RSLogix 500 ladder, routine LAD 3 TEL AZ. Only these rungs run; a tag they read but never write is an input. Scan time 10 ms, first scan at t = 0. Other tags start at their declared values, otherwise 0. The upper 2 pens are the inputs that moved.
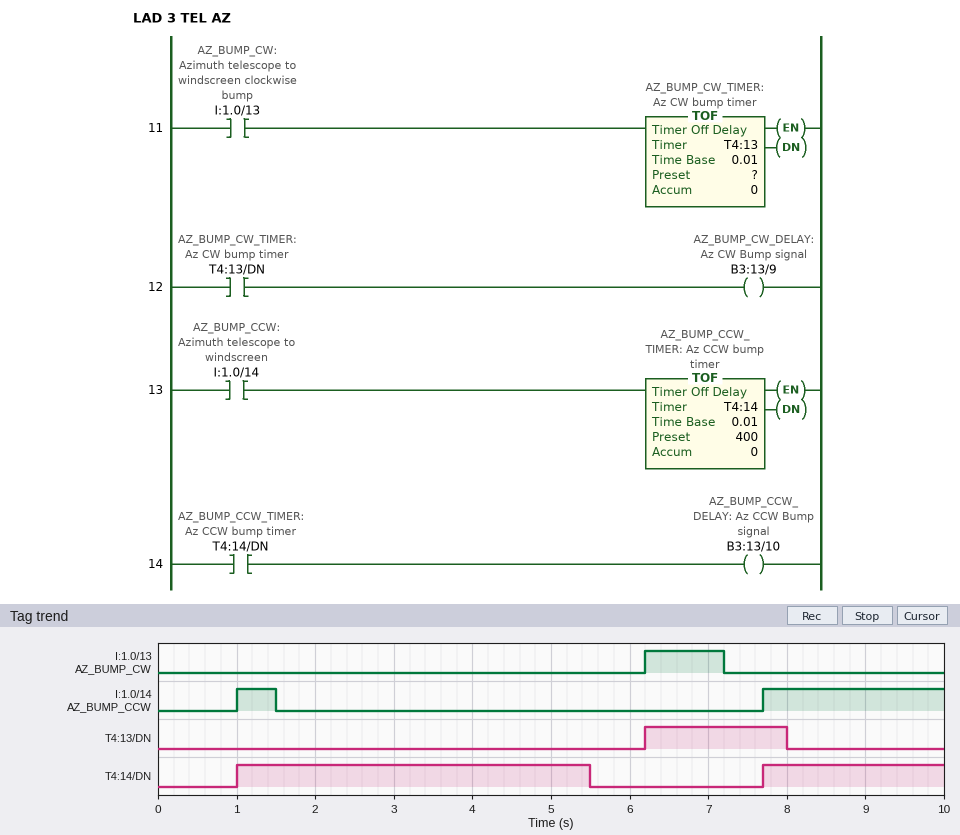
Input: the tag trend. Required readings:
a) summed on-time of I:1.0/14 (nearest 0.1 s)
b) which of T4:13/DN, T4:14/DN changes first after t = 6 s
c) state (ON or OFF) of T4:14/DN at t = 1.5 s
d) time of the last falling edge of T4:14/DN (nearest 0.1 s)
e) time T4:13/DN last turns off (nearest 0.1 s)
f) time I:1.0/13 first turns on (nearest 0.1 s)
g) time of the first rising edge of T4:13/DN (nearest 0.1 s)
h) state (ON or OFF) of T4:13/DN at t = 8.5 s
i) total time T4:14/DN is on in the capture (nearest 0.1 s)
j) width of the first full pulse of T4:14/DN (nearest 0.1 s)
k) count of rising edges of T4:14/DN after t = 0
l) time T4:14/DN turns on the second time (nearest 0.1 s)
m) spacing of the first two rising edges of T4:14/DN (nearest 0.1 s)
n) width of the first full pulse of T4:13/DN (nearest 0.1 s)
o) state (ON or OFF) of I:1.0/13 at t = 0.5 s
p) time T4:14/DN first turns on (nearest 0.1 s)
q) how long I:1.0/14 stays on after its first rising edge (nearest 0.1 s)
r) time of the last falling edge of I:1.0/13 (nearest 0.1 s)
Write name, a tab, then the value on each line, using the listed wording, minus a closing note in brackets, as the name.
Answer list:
summed on-time of I:1.0/14	2.8 s
which of T4:13/DN, T4:14/DN changes first after t = 6 s	T4:13/DN
state (ON or OFF) of T4:14/DN at t = 1.5 s	ON
time of the last falling edge of T4:14/DN	5.5 s
time T4:13/DN last turns off	8.0 s
time I:1.0/13 first turns on	6.2 s
time of the first rising edge of T4:13/DN	6.2 s
state (ON or OFF) of T4:13/DN at t = 8.5 s	OFF
total time T4:14/DN is on in the capture	6.8 s
width of the first full pulse of T4:14/DN	4.5 s
count of rising edges of T4:14/DN after t = 0	2
time T4:14/DN turns on the second time	7.7 s
spacing of the first two rising edges of T4:14/DN	6.7 s
width of the first full pulse of T4:13/DN	1.8 s
state (ON or OFF) of I:1.0/13 at t = 0.5 s	OFF
time T4:14/DN first turns on	1.0 s
how long I:1.0/14 stays on after its first rising edge	0.5 s
time of the last falling edge of I:1.0/13	7.2 s
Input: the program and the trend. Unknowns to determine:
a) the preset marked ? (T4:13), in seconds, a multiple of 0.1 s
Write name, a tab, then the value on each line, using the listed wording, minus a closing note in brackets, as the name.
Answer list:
the preset marked ? (T4:13), in seconds, a multiple of 0.1 s	0.8 s
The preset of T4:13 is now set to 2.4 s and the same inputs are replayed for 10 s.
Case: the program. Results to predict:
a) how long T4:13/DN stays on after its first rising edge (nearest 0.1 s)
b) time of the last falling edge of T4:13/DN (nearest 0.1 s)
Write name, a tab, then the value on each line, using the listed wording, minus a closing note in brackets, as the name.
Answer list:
how long T4:13/DN stays on after its first rising edge	3.4 s
time of the last falling edge of T4:13/DN	9.6 s
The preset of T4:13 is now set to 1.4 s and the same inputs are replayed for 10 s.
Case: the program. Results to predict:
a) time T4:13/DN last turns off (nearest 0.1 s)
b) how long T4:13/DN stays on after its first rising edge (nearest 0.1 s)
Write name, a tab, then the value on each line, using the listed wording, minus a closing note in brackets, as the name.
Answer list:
time T4:13/DN last turns off	8.6 s
how long T4:13/DN stays on after its first rising edge	2.4 s
